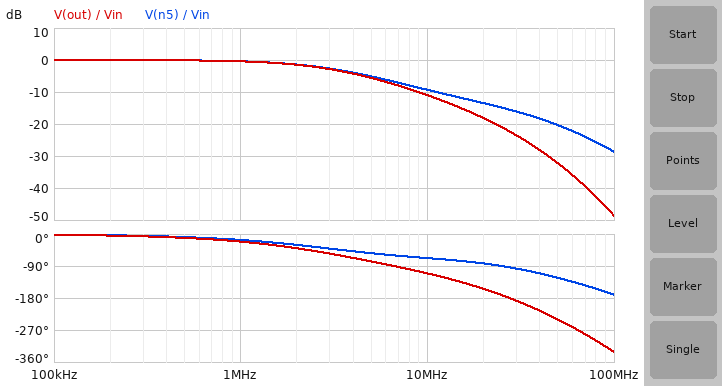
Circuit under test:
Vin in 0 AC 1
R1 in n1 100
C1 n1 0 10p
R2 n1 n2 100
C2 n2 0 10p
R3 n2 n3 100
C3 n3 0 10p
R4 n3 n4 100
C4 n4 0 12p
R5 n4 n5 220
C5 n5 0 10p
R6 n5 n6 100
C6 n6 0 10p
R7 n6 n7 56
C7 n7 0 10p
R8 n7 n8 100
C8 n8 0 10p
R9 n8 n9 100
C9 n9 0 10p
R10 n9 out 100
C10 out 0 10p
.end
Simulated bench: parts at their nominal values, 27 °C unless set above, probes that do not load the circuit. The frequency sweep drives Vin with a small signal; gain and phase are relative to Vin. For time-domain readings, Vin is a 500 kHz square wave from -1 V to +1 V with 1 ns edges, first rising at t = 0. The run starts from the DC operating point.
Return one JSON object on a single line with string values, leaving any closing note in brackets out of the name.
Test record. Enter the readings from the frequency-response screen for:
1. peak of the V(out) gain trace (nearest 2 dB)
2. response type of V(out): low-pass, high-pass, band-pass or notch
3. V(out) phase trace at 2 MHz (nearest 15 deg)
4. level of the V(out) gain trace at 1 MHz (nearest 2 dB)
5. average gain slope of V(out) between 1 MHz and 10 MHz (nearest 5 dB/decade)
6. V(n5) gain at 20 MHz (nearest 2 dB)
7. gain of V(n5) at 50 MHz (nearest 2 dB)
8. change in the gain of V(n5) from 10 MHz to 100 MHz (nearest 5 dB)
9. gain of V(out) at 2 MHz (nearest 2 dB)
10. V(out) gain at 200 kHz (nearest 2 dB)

{"peak of the V(out) gain trace": "0 dB", "response type of V(out): low-pass, high-pass, band-pass or notch": "low-pass", "V(out) phase trace at 2 MHz": "-45 deg", "level of the V(out) gain trace at 1 MHz": "0 dB", "average gain slope of V(out) between 1 MHz and 10 MHz": "-10 dB/decade", "V(n5) gain at 20 MHz": "-14 dB", "gain of V(n5) at 50 MHz": "-20 dB", "change in the gain of V(n5) from 10 MHz to 100 MHz": "-20 dB", "gain of V(out) at 2 MHz": "-2 dB", "V(out) gain at 200 kHz": "0 dB"}
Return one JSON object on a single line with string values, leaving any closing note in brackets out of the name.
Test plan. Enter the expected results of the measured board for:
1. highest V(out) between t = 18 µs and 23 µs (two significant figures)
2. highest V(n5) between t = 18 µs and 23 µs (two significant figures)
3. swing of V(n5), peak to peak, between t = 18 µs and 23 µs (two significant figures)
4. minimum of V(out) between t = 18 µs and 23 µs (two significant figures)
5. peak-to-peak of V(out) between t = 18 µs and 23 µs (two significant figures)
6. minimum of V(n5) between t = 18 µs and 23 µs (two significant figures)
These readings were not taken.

{"highest V(out) between t = 18 µs and 23 µs": "1.0 V", "highest V(n5) between t = 18 µs and 23 µs": "1.0 V", "swing of V(n5), peak to peak, between t = 18 µs and 23 µs": "2.0 V", "minimum of V(out) between t = 18 µs and 23 µs": "-1.0 V", "peak-to-peak of V(out) between t = 18 µs and 23 µs": "2.0 V", "minimum of V(n5) between t = 18 µs and 23 µs": "-1.0 V"}
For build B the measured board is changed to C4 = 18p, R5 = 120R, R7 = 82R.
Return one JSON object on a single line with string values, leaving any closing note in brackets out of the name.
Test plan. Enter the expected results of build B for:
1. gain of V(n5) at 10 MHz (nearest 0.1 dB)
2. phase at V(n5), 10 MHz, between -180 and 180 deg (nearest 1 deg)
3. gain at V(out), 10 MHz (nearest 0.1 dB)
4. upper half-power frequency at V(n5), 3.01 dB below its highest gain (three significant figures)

{"gain of V(n5) at 10 MHz": "-8.7 dB", "phase at V(n5), 10 MHz, between -180 and 180 deg": "-65 deg", "gain at V(out), 10 MHz": "-10.6 dB", "upper half-power frequency at V(n5), 3.01 dB below its highest gain": "3.51 MHz"}
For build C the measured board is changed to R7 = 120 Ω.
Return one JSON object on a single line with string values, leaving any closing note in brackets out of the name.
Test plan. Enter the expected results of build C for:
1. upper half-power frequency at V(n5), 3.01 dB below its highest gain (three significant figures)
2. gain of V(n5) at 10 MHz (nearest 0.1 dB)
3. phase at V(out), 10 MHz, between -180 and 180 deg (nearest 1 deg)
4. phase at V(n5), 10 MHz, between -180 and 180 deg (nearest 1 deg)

{"upper half-power frequency at V(n5), 3.01 dB below its highest gain": "3.21 MHz", "gain of V(n5) at 10 MHz": "-9.1 dB", "phase at V(out), 10 MHz, between -180 and 180 deg": "-114 deg", "phase at V(n5), 10 MHz, between -180 and 180 deg": "-65 deg"}
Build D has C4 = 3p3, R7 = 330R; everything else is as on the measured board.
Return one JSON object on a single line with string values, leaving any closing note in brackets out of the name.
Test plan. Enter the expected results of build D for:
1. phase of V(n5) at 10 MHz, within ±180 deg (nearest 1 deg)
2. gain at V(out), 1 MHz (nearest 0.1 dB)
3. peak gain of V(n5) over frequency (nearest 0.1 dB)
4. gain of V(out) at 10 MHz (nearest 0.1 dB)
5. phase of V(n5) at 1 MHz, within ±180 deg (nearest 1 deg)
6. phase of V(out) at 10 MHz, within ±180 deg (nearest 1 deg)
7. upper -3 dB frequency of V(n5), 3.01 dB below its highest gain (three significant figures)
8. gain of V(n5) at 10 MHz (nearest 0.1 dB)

{"phase of V(n5) at 10 MHz, within ±180 deg": "-53 deg", "gain at V(out), 1 MHz": "-0.5 dB", "peak gain of V(n5) over frequency": "0 dB", "gain of V(out) at 10 MHz": "-12.1 dB", "phase of V(n5) at 1 MHz, within ±180 deg": "-15 deg", "phase of V(out) at 10 MHz, within ±180 deg": "-117 deg", "upper -3 dB frequency of V(n5), 3.01 dB below its highest gain": "3.25 MHz", "gain of V(n5) at 10 MHz": "-7.6 dB"}
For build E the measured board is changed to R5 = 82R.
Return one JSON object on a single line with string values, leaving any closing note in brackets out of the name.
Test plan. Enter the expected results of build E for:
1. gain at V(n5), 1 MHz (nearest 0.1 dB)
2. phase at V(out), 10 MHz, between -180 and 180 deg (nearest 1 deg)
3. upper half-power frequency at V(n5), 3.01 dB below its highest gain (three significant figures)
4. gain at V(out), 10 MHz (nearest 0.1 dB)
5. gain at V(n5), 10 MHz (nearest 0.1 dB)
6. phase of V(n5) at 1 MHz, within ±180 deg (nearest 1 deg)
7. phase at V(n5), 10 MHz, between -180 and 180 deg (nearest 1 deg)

{"gain at V(n5), 1 MHz": "-0.3 dB", "phase at V(out), 10 MHz, between -180 and 180 deg": "-104 deg", "upper half-power frequency at V(n5), 3.01 dB below its highest gain": "3.87 MHz", "gain at V(out), 10 MHz": "-9.7 dB", "gain at V(n5), 10 MHz": "-8.0 dB", "phase of V(n5) at 1 MHz, within ±180 deg": "-14 deg", "phase at V(n5), 10 MHz, between -180 and 180 deg": "-61 deg"}
